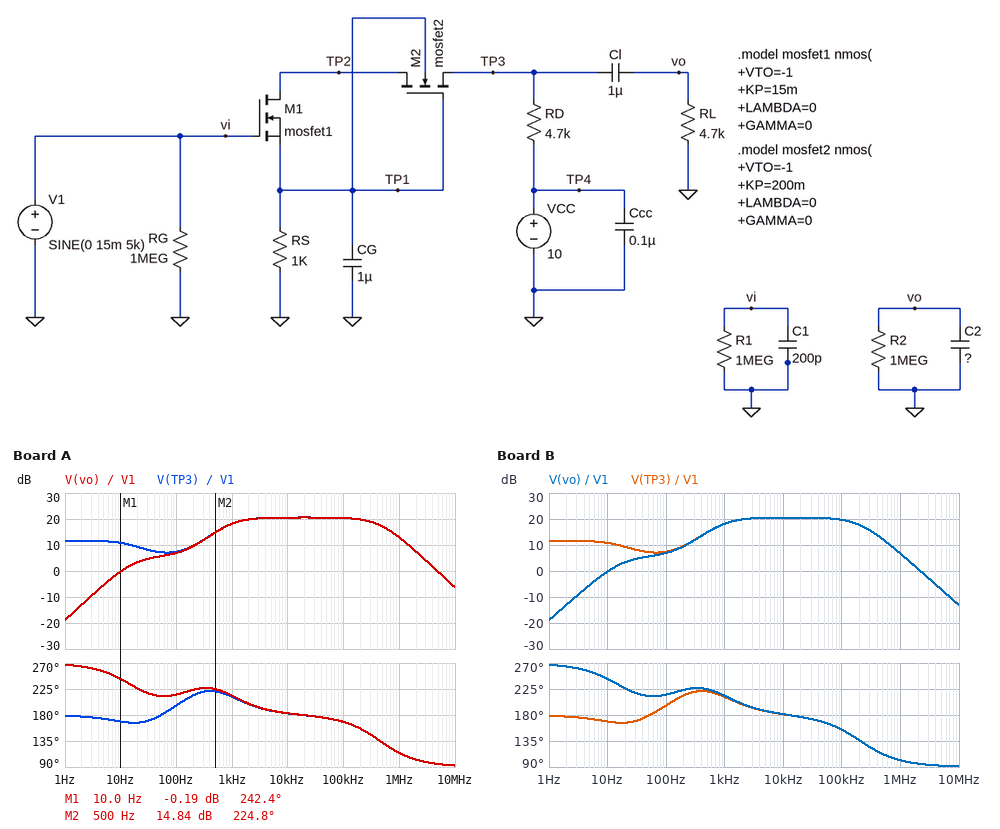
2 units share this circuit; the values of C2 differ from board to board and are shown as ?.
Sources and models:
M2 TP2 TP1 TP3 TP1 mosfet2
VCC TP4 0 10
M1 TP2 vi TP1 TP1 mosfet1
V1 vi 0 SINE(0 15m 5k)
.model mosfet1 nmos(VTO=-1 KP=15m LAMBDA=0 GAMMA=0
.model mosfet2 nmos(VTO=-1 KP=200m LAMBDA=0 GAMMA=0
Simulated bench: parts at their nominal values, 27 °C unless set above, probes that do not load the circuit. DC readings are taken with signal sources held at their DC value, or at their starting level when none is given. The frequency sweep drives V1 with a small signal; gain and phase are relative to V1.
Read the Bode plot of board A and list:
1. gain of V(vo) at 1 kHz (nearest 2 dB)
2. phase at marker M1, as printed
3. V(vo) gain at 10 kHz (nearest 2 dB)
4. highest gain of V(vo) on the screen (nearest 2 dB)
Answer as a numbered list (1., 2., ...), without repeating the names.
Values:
1. 18 dB
2. 242.4 deg
3. 20 dB
4. 20 dB
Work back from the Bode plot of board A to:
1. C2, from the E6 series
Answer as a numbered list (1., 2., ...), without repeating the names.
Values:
1. 150 pF
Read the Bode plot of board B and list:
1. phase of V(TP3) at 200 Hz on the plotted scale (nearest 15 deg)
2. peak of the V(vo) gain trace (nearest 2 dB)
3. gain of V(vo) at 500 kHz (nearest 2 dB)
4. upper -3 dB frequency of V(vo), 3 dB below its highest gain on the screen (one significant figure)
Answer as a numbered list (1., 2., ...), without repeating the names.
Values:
1. 210 deg
2. 20 dB
3. 12 dB
4. 200 kHz
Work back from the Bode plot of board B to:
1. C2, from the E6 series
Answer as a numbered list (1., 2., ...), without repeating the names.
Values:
1. 330 pF
